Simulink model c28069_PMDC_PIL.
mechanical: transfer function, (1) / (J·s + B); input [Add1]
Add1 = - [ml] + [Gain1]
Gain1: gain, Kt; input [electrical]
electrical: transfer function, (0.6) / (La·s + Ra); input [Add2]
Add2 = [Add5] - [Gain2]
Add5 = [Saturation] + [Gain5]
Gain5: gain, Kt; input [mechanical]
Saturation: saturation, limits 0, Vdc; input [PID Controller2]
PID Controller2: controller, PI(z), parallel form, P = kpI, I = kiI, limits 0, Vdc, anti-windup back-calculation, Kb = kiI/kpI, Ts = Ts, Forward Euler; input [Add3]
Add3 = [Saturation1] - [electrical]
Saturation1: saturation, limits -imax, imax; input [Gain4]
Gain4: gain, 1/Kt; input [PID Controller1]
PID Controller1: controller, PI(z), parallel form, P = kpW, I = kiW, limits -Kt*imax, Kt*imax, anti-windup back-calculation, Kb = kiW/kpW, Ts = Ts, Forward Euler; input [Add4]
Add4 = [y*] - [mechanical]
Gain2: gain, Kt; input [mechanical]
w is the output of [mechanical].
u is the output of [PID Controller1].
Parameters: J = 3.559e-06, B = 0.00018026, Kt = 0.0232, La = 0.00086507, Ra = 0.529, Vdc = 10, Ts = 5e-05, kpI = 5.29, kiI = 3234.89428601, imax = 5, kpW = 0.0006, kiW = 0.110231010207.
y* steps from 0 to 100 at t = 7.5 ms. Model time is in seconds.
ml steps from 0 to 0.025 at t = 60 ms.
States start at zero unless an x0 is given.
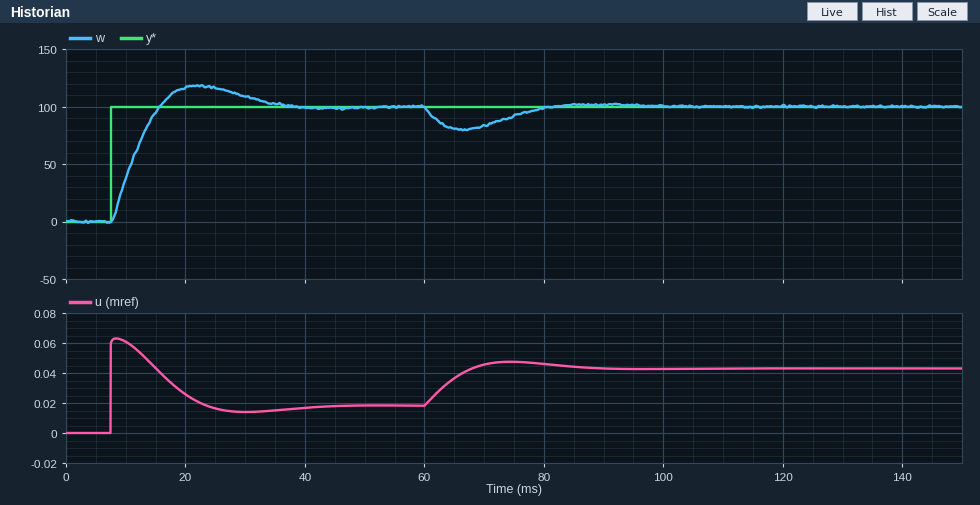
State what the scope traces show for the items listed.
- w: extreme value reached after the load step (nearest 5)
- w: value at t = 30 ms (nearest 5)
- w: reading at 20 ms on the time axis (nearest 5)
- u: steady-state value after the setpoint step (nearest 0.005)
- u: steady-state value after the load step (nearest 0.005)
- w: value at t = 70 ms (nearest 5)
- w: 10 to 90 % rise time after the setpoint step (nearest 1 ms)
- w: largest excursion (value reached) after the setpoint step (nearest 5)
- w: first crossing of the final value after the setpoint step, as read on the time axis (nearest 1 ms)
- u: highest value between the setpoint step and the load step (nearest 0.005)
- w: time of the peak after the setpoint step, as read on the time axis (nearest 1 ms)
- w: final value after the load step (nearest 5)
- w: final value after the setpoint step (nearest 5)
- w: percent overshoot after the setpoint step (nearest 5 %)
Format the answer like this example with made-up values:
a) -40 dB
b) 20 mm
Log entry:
a) 80
b) 110
c) 115
d) 0.020
e) 0.045
f) 85
g) 6 ms
h) 120
i) 16 ms
j) 0.065
k) 22 ms
l) 100
m) 100
n) 20 %
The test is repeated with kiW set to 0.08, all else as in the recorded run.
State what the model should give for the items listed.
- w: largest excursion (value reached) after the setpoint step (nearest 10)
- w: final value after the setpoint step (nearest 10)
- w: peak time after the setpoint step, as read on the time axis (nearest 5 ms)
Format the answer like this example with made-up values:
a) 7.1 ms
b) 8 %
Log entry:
a) 110
b) 100
c) 25 ms
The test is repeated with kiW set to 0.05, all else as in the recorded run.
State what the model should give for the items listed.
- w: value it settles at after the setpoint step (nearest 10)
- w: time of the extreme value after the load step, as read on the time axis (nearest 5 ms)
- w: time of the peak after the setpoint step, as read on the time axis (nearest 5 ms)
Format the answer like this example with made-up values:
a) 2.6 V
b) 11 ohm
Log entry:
a) 100
b) 70 ms
c) 30 ms
